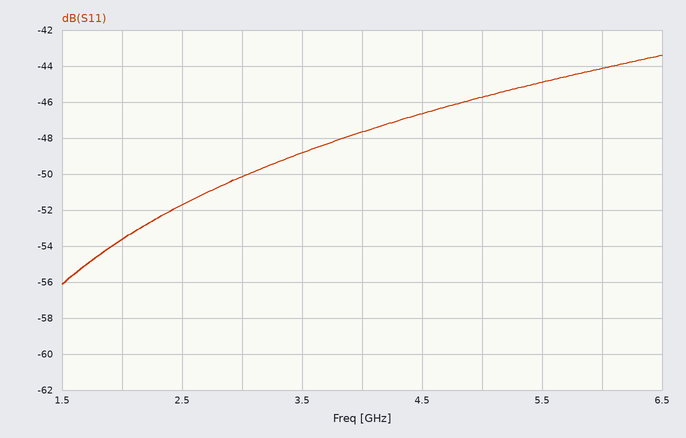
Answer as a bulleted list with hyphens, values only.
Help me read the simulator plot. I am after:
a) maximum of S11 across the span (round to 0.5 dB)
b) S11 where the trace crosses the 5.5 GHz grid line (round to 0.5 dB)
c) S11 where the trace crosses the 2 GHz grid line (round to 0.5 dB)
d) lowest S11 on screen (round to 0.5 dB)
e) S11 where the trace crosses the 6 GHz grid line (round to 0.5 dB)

- -43.5 dB
- -45.0 dB
- -53.5 dB
- -56.0 dB
- -44.0 dB
